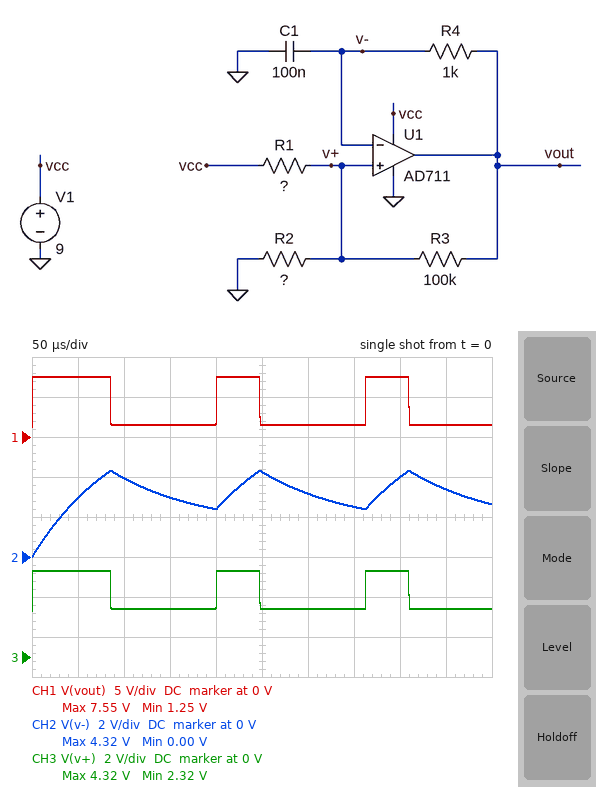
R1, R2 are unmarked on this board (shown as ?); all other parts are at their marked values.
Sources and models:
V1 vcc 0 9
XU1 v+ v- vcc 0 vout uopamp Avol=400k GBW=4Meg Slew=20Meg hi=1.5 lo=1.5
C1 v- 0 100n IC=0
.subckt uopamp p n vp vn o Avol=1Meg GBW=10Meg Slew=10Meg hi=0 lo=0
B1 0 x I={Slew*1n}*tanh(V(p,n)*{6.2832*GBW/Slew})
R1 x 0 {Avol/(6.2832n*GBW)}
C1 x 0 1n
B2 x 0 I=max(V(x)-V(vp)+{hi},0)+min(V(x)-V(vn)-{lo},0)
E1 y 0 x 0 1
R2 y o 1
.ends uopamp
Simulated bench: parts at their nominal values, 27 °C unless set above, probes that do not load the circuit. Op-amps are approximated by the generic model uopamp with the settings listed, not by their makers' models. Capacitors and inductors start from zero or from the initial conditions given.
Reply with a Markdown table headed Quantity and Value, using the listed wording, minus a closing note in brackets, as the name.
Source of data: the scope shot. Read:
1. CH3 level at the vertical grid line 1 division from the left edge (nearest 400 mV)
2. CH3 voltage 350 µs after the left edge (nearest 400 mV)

| Quantity | Value |
|---|---|
| CH3 level at the vertical grid line 1 division from the left edge | 4.4 V |
| CH3 voltage 350 µs after the left edge | 2.4 V |
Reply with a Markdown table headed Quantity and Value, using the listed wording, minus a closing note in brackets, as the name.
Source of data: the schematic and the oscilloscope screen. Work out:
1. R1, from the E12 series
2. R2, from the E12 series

| Quantity | Value |
|---|---|
| R1, from the E12 series | 150 kΩ |
| R2, from the E12 series | 68 kΩ |
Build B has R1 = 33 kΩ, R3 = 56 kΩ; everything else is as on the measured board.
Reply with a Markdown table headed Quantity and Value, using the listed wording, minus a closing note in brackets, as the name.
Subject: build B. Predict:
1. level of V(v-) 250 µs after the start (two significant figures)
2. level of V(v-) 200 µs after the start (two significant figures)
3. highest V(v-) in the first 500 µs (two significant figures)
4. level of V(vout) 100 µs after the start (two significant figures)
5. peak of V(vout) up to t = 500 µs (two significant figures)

| Quantity | Value |
|---|---|
| level of V(v-) 250 µs after the start | 5.0 V |
| level of V(v-) 200 µs after the start | 6.4 V |
| highest V(v-) in the first 500 µs | 6.5 V |
| level of V(vout) 100 µs after the start | 7.5 V |
| peak of V(vout) up to t = 500 µs | 7.5 V |
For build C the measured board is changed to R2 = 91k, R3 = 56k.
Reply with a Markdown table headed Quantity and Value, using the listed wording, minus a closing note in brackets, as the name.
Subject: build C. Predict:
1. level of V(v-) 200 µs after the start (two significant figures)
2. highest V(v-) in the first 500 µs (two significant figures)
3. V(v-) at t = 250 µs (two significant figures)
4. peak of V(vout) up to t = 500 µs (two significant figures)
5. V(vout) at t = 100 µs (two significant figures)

| Quantity | Value |
|---|---|
| level of V(v-) 200 µs after the start | 3.5 V |
| highest V(v-) in the first 500 µs | 5.5 V |
| V(v-) at t = 250 µs | 2.7 V |
| peak of V(vout) up to t = 500 µs | 7.5 V |
| V(vout) at t = 100 µs | 7.5 V |
